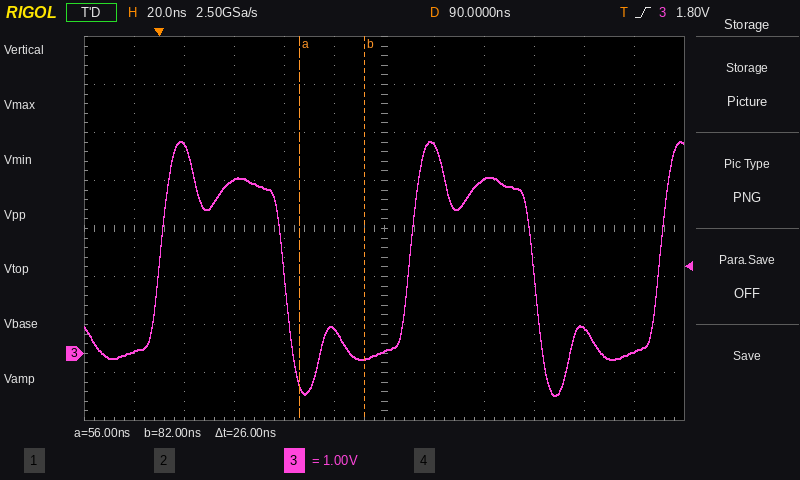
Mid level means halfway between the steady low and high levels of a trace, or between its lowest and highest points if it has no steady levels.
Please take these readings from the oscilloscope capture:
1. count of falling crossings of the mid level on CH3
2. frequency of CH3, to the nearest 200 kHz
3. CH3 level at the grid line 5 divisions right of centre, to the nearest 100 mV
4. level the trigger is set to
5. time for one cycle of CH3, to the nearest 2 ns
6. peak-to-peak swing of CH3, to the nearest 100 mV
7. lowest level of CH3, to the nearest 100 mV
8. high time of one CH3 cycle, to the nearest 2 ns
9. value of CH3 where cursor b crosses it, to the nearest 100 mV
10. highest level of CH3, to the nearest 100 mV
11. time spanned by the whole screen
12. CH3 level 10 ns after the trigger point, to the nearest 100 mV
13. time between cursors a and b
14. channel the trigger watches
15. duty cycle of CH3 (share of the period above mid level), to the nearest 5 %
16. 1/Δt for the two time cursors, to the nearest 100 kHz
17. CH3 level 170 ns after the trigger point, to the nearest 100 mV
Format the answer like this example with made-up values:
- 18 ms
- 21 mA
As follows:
- 2
- 10.0 MHz
- 0.0 V
- 1.80 V
- 100 ns
- 5.3 V
- -900 mV
- 50 ns
- -100 mV
- 4.4 V
- 240 ns
- 4.3 V
- 26 ns
- CH3
- 50 %
- 38.5 MHz
- 500 mV
